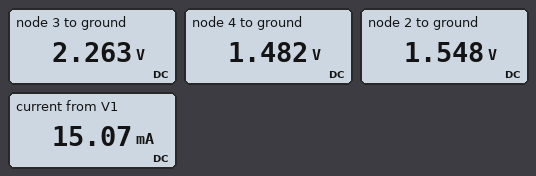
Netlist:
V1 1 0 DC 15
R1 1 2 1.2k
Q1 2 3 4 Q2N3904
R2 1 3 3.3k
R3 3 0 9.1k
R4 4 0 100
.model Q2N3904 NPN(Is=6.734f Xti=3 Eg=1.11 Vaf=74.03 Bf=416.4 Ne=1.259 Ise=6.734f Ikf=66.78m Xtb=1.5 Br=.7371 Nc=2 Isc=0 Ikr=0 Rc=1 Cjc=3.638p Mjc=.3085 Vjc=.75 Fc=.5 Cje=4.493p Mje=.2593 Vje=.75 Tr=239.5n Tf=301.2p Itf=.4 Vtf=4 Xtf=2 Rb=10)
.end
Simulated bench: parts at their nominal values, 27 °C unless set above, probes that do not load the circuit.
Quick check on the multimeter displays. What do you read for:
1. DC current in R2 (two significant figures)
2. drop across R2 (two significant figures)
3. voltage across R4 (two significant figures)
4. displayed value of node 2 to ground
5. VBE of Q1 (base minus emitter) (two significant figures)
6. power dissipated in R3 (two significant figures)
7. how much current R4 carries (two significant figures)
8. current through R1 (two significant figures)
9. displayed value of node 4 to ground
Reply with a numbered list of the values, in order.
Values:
1. 3.9 mA
2. 13 V
3. 1.5 V
4. 1.548 V
5. 780 mV
6. 560 µW
7. 15 mA
8. 11 mA
9. 1.482 V
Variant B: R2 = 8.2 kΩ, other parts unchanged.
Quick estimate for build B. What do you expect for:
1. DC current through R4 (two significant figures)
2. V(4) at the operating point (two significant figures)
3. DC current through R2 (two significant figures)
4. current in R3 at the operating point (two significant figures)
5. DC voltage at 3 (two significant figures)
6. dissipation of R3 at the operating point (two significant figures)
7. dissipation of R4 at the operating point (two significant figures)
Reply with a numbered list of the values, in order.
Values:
1. 13 mA
2. 1.3 V
3. 1.6 mA
4. 220 µA
5. 2.0 V
6. 450 µW
7. 16 mW
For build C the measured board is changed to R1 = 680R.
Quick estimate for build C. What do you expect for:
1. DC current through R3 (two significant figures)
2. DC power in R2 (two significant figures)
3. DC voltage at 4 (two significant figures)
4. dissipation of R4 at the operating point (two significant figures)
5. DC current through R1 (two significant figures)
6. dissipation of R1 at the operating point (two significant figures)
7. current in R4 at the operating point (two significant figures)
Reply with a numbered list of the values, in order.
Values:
1. 330 µA
2. 44 mW
3. 2.2 V
4. 48 mW
5. 19 mA
6. 240 mW
7. 22 mA
